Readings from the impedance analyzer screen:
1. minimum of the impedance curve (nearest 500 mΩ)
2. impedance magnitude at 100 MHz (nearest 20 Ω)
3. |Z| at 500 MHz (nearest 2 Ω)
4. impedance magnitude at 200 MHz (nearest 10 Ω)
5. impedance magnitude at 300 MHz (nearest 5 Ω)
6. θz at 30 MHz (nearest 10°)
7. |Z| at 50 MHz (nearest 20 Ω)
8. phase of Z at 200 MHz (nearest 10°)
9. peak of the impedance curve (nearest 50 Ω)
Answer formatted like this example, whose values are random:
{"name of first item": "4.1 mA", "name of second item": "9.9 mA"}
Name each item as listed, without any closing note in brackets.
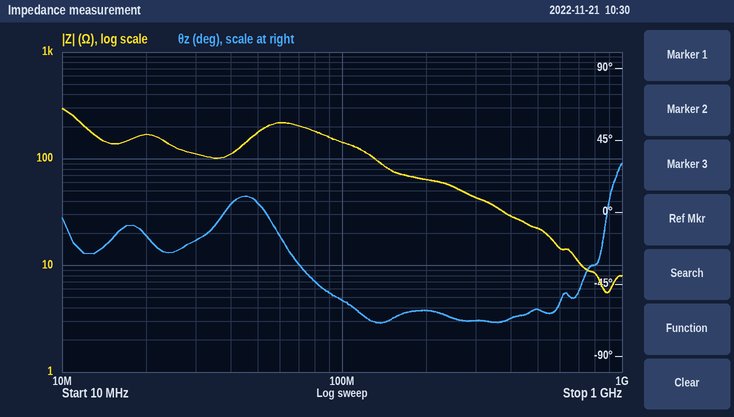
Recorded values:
{"minimum of the impedance curve": "5.5 Ω", "impedance magnitude at 100 MHz": "140 Ω", "|Z| at 500 MHz": "22 Ω", "impedance magnitude at 200 MHz": "60 Ω", "impedance magnitude at 300 MHz": "45 Ω", "θz at 30 MHz": "-20°", "|Z| at 50 MHz": "180 Ω", "phase of Z at 200 MHz": "-60°", "peak of the impedance curve": "300 Ω"}
